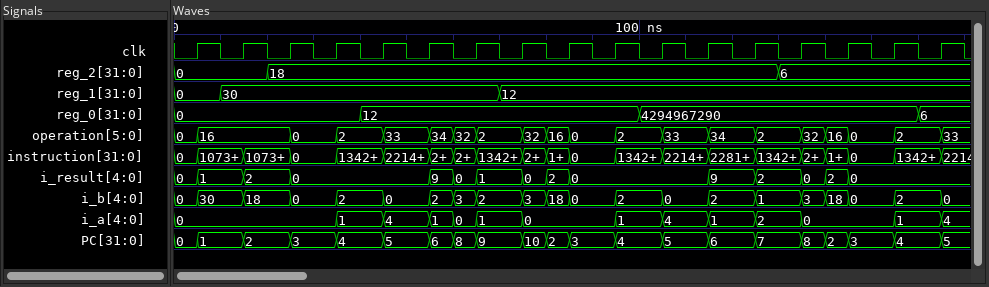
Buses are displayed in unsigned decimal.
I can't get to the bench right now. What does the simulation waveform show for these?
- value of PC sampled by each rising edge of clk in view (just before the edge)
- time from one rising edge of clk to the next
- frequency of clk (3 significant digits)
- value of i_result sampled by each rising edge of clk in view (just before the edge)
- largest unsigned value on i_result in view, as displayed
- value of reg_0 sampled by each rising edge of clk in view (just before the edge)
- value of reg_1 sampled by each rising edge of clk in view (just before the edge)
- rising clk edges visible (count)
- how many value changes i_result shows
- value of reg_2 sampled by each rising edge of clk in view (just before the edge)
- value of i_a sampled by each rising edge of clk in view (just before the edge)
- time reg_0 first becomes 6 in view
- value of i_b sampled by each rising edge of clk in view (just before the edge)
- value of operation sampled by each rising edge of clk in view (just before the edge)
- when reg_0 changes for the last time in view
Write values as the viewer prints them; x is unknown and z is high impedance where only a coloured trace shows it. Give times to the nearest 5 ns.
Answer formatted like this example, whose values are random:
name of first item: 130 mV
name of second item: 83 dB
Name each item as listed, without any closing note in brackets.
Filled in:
value of PC sampled by each rising edge of clk in view: 0, 1, 2, 3, 4, 5, 8, 9, 2, 3, 4, 5, 6, 7, 2, 3, 4
time from one rising edge of clk to the next: 10 ns
frequency of clk: 100 MHz
value of i_result sampled by each rising edge of clk in view: 0, 1, 2, 0, 0, 0, 0, 1, 2, 0, 0, 0, 9, 2, 2, 0, 0
largest unsigned value on i_result in view, as displayed: 9
value of reg_0 sampled by each rising edge of clk in view: 0, 0, 0, 0, 12, 12, 12, 12, 12, 12, 4294967290, 4294967290, 4294967290, 4294967290, 4294967290, 4294967290, 6
value of reg_1 sampled by each rising edge of clk in view: 0, 30, 30, 30, 30, 30, 30, 12, 12, 12, 12, 12, 12, 12, 12, 12, 12
rising clk edges visible: 17
how many value changes i_result shows: 14
value of reg_2 sampled by each rising edge of clk in view: 0, 0, 18, 18, 18, 18, 18, 18, 18, 18, 18, 18, 18, 6, 6, 6, 6
value of i_a sampled by each rising edge of clk in view: 0, 0, 0, 0, 1, 4, 0, 1, 0, 0, 1, 4, 1, 2, 0, 0, 1
time reg_0 first becomes 6 in view: 160 ns
value of i_b sampled by each rising edge of clk in view: 0, 30, 18, 0, 2, 0, 3, 2, 18, 0, 2, 0, 2, 1, 18, 0, 2
value of operation sampled by each rising edge of clk in view: 0, 16, 16, 0, 2, 33, 32, 2, 16, 0, 2, 33, 34, 2, 16, 0, 2
when reg_0 changes for the last time in view: 160 ns
